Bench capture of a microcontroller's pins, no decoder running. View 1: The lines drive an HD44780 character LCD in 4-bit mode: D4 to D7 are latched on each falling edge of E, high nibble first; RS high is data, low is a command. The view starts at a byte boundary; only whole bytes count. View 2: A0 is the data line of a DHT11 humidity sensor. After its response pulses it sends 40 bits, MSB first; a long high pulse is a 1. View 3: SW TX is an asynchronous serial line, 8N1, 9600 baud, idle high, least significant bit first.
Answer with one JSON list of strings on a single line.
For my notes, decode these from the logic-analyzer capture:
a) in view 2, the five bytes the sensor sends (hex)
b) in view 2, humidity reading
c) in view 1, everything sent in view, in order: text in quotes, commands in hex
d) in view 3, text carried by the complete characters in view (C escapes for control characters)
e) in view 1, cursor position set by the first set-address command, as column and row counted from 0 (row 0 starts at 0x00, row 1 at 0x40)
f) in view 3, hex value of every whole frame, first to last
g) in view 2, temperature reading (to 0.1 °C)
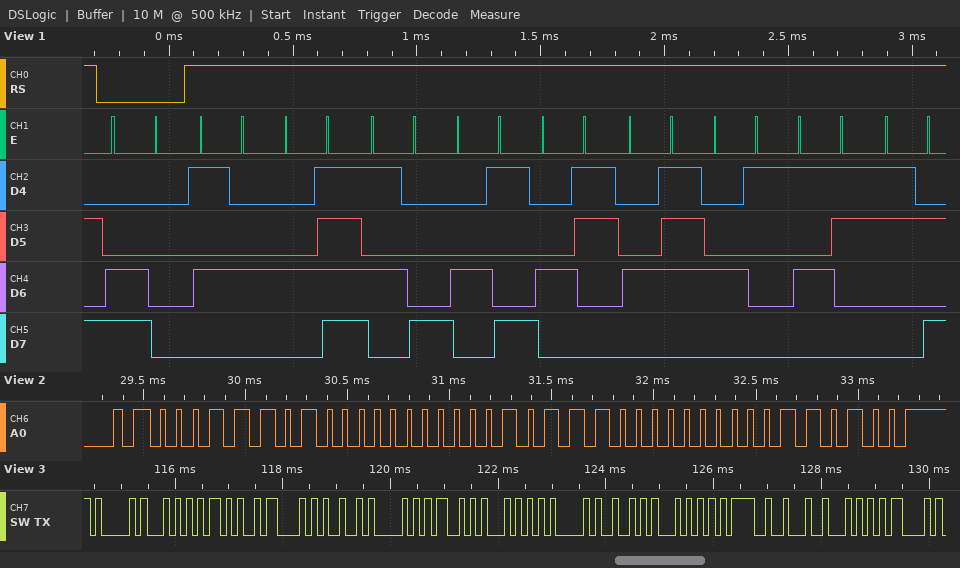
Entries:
["1D 00 17 00 34", "29 %", "0xC0 \"TOXICGAS:\"", "\"AT+CIPSTART=\\\"TC\"", "column 0, row 1", "41 54 2B 43 49 50 53 54 41 52 54 3D 22 54 43", "23.0 °C"]
